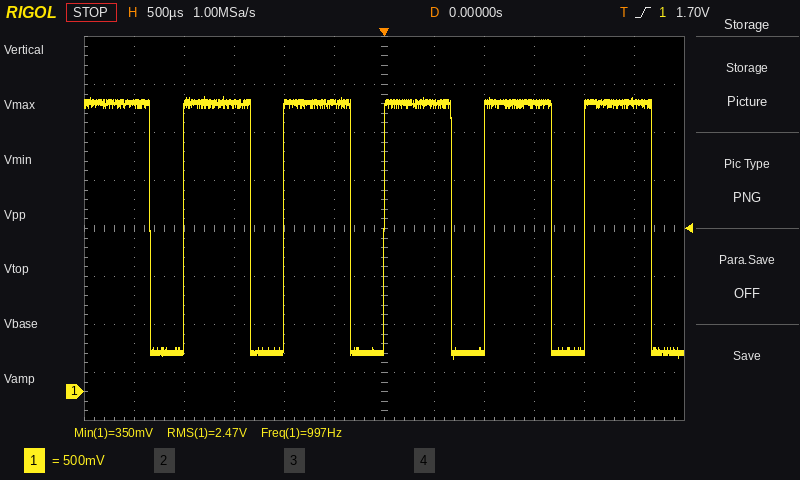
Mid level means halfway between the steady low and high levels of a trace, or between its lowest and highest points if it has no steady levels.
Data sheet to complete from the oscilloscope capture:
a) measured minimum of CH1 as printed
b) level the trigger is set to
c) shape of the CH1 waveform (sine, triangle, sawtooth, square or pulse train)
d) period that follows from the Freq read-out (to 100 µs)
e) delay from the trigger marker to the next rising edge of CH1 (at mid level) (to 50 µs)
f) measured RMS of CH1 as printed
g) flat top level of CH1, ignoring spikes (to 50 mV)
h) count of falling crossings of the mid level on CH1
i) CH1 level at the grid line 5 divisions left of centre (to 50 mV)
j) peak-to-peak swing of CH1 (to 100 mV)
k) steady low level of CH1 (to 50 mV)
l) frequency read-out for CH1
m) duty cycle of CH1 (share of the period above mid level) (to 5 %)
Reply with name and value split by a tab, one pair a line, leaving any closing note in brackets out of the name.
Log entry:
measured minimum of CH1 as printed	350 mV
level the trigger is set to	1.70 V
shape of the CH1 waveform	pulse train
period that follows from the Freq read-out	1.0 ms
delay from the trigger marker to the next rising edge of CH1 (at mid level)	1.00 ms
measured RMS of CH1 as printed	2.47 V
flat top level of CH1, ignoring spikes	3.00 V
count of falling crossings of the mid level on CH1	6
CH1 level at the grid line 5 divisions left of centre	3.00 V
peak-to-peak swing of CH1	2.70 V
steady low level of CH1	400 mV
frequency read-out for CH1	997 Hz
duty cycle of CH1 (share of the period above mid level)	65 %
